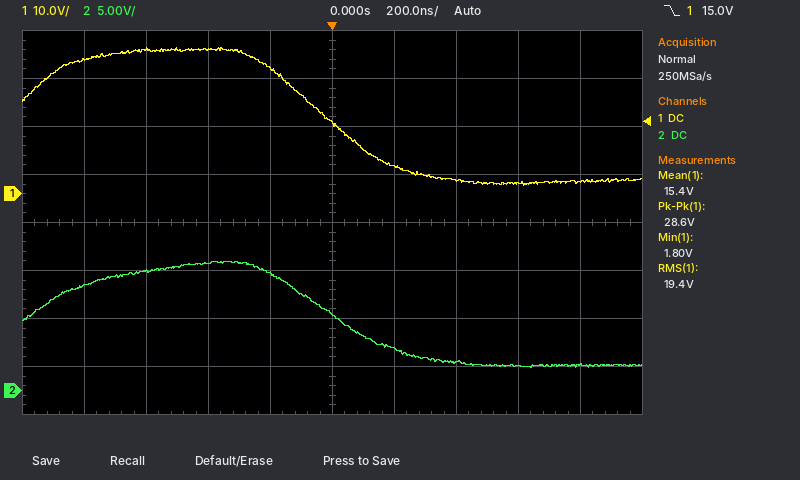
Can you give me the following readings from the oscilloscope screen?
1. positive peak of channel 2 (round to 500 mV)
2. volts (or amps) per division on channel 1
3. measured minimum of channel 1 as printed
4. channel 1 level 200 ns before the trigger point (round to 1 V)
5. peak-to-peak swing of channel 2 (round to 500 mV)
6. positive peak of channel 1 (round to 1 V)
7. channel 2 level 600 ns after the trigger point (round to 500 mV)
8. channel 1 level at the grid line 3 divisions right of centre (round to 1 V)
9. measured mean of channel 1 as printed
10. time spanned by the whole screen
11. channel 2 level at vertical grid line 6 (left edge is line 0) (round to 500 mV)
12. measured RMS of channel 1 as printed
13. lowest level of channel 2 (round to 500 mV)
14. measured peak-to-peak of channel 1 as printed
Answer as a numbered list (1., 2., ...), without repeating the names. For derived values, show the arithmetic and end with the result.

1. 13.5 V
2. 10 V
3. 1.80 V
4. 26 V
5. 13.5 V − (2.5 V) = 11.0 V
6. 30 V
7. 2.5 V
8. 2 V
9. 15.4 V
10. 2 µs
11. 4.5 V
12. 19.4 V
13. 2.5 V
14. 28.6 V
